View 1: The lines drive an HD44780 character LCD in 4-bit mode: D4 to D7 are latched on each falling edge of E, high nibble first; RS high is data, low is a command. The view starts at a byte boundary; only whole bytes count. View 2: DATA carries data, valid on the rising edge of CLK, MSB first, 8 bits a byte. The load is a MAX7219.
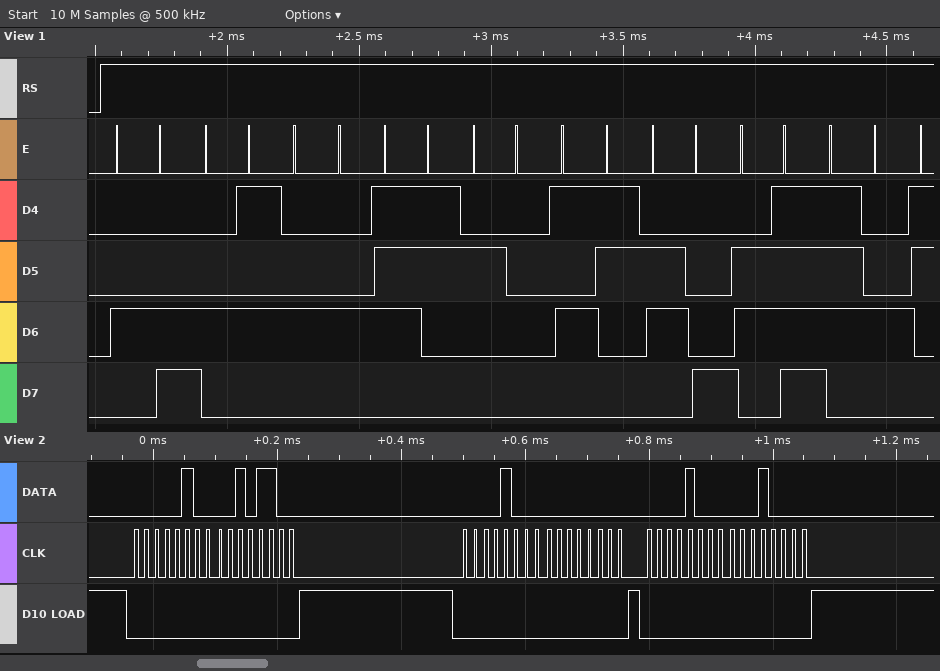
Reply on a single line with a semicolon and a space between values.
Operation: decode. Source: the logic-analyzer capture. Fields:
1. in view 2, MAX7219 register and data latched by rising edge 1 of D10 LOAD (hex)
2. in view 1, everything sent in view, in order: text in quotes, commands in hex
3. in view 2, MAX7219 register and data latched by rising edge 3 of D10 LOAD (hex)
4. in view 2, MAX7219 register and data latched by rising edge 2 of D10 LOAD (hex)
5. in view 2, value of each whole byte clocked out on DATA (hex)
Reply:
register 0x4, data 0x2C; "LEDs Shot"; register 0x8, data 0x10; register 0x8, data 0x00; 04 2C 08 00 08 10
